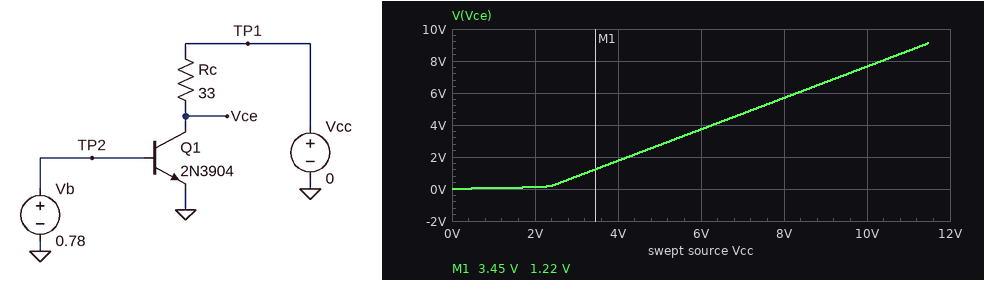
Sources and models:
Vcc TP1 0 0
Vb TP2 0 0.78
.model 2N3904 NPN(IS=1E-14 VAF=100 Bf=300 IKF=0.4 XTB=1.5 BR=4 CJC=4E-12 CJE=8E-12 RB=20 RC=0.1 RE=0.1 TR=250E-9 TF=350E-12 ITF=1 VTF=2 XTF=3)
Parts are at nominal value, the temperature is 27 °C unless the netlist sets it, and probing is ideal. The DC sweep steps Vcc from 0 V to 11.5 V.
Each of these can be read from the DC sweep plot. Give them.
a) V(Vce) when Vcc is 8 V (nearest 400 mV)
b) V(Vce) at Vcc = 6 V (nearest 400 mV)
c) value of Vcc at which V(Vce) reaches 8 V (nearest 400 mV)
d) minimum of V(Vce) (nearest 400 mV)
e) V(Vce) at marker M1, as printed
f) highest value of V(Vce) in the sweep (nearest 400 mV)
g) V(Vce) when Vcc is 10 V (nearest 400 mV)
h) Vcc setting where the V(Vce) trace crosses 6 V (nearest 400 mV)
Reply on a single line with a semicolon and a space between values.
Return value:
5.6 V; 3.6 V; 10.4 V; 0 V; 1.22 V; 9.2 V; 7.6 V; 8.4 V
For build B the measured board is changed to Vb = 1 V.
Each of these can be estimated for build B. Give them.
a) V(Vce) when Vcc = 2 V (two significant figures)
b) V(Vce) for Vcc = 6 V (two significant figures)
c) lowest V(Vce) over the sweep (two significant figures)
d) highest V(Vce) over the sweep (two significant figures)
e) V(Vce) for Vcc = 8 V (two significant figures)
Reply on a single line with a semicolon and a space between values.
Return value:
43 mV; 97 mV; 7.5 mV; 160 mV; 120 mV
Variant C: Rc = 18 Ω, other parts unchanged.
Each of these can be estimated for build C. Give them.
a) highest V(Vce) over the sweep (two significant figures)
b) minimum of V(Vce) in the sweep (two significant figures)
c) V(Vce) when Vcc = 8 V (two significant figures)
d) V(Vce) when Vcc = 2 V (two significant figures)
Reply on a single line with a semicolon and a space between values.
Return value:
10 V; 5.6 mV; 6.7 V; 790 mV
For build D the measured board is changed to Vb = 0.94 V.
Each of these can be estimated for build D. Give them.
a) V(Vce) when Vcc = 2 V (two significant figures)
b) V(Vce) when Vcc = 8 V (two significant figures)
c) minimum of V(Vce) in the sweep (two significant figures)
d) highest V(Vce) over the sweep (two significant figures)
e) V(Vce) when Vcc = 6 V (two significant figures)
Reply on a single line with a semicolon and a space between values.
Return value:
47 mV; 130 mV; 7.1 mV; 180 mV; 110 mV
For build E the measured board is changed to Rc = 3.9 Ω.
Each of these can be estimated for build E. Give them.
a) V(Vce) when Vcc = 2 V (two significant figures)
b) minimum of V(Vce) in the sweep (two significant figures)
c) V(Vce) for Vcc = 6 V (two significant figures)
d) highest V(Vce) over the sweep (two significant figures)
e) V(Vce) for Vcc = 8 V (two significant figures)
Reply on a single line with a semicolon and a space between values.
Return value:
1.7 V; 4.0 mV; 5.7 V; 11 V; 7.7 V
